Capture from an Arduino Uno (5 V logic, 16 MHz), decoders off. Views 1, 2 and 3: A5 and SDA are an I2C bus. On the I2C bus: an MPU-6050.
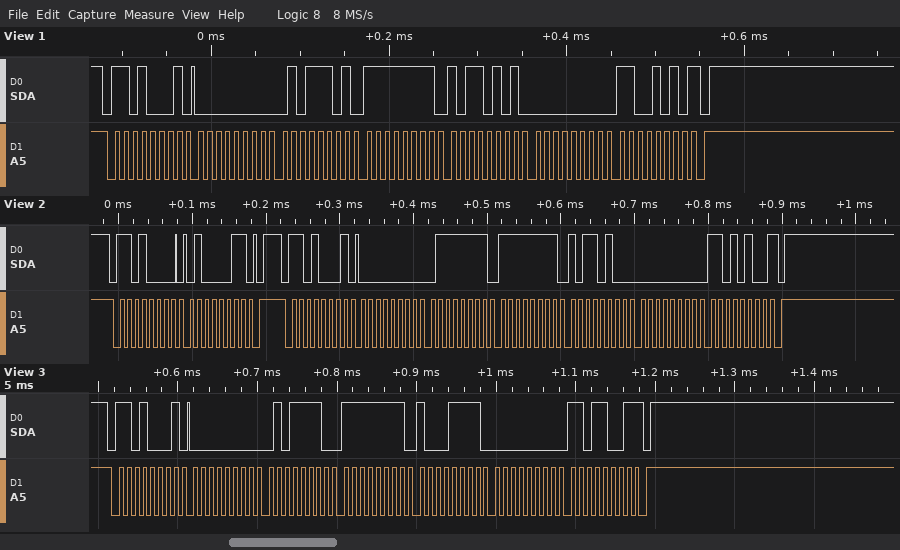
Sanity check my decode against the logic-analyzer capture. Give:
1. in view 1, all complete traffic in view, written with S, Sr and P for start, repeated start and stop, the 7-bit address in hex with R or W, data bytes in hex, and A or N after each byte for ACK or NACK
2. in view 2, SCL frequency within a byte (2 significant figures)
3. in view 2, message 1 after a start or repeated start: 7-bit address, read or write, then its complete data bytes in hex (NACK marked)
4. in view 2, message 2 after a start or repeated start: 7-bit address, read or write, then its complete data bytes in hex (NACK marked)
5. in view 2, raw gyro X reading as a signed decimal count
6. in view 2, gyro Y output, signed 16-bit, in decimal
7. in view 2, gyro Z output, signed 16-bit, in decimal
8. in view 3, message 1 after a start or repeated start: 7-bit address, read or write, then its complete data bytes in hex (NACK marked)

S 68R A 00 A 5D A FF A B5 A 00 A CA N P
100 kHz
0x68 write: 43
0x68 read: 00 7F FF B4 00 D4 NACK
127
-76
212
0x68 read: 00 5E FF 8F 00 D9 NACK
